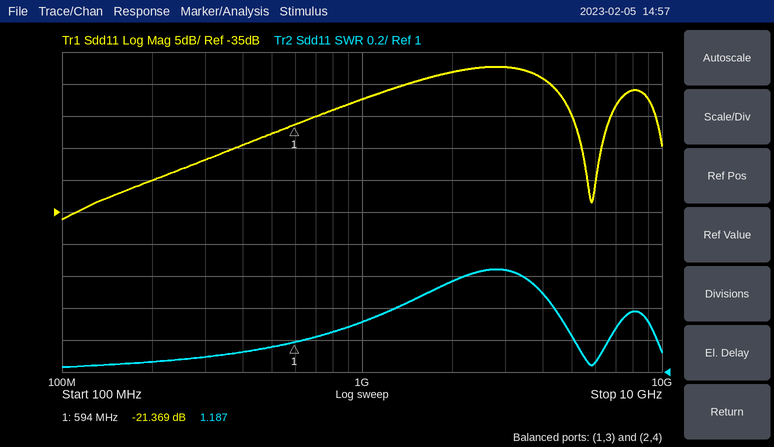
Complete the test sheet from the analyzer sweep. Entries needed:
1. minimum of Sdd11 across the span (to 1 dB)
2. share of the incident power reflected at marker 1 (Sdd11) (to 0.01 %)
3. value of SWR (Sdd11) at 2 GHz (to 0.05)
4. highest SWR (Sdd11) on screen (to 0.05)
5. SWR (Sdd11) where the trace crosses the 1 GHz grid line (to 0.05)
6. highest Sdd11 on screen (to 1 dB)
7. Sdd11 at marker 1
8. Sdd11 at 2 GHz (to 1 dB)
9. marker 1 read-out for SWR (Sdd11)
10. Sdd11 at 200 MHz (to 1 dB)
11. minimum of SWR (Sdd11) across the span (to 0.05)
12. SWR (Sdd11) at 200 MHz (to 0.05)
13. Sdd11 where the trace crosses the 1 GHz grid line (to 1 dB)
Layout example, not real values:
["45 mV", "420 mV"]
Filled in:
["-36 dB", "0.73 %", "1.55", "1.65", "1.30", "-12 dB", "-21.369 dB", "-13 dB", "1.187", "-30 dB", "1.05", "1.05", "-17 dB"]
